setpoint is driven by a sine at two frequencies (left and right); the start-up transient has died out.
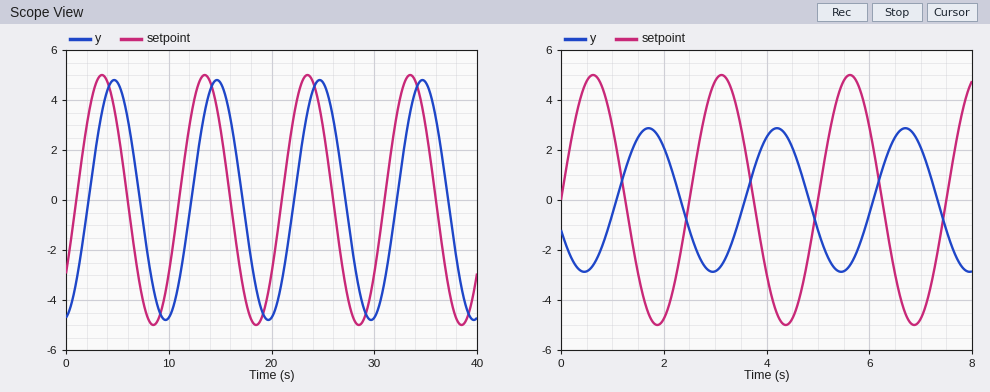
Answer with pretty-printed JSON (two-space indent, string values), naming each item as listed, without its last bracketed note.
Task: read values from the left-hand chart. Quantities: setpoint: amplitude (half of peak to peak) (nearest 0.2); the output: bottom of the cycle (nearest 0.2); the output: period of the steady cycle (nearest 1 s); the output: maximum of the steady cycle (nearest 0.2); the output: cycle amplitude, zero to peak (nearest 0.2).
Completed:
{
  "setpoint: amplitude (half of peak to peak)": "5.0",
  "the output: bottom of the cycle": "-4.8",
  "the output: period of the steady cycle": "10 s",
  "the output: maximum of the steady cycle": "4.8",
  "the output: cycle amplitude, zero to peak": "4.8"
}
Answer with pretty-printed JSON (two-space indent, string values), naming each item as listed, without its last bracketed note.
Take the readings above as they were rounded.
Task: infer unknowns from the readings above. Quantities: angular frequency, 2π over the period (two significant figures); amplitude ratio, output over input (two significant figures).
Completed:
{
  "angular frequency, 2π over the period": "0.63 rad/s",
  "amplitude ratio, output over input": "0.96"
}
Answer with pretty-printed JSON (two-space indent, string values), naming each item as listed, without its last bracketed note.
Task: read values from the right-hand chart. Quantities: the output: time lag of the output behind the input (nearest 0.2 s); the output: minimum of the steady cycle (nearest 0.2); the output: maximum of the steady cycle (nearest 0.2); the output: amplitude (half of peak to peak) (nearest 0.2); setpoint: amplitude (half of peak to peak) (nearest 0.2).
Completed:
{
  "the output: time lag of the output behind the input": "1.0 s",
  "the output: minimum of the steady cycle": "-2.8",
  "the output: maximum of the steady cycle": "2.8",
  "the output: amplitude (half of peak to peak)": "2.8",
  "setpoint: amplitude (half of peak to peak)": "5.0"
}
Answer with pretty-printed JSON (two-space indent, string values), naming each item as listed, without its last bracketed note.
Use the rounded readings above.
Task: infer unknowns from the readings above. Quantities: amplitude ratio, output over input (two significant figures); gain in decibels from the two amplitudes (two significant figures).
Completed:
{
  "amplitude ratio, output over input": "0.56",
  "gain in decibels from the two amplitudes": "-5.0 dB"
}
